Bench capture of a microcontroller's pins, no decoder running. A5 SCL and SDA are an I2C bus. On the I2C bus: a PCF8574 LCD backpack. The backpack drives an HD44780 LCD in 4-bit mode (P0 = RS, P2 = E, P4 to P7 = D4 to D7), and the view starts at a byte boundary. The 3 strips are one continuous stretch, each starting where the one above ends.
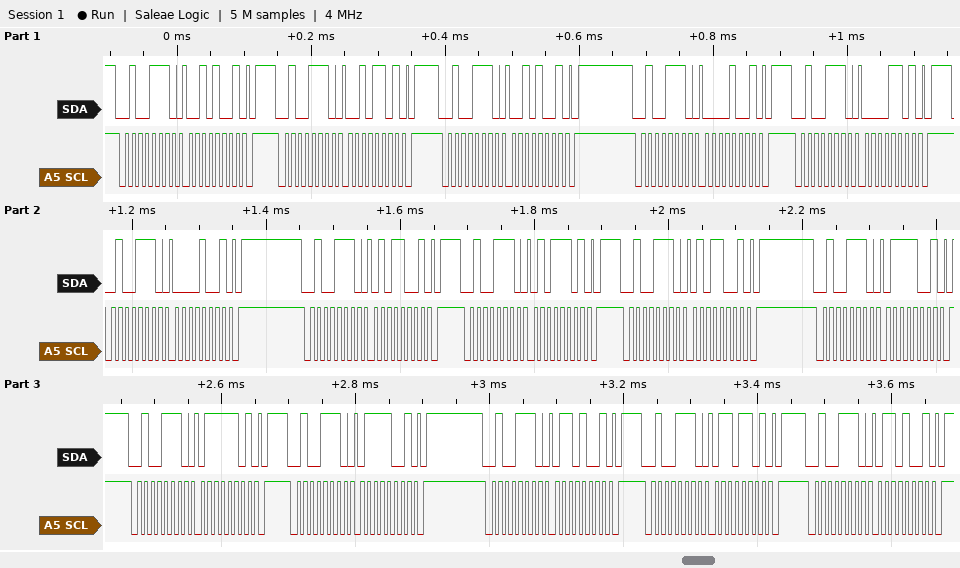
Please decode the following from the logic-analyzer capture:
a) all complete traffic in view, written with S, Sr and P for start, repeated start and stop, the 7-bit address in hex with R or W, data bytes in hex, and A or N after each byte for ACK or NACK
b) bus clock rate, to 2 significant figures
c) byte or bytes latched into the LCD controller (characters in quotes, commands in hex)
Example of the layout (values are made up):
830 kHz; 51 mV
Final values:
S 27W A 29 A P S 27W A 2D A P S 27W A 29 A P S 27W A 09 A P S 27W A 0D A P S 27W A 09 A P S 27W A 59 A P S 27W A 5D A P S 27W A 59 A P S 27W A 79 A P S 27W A 7D A P S 27W A 79 A P S 27W A 69 A P S 27W A 6D A P S 27W A 69 A P; 100 kHz; ' ' 'W'
